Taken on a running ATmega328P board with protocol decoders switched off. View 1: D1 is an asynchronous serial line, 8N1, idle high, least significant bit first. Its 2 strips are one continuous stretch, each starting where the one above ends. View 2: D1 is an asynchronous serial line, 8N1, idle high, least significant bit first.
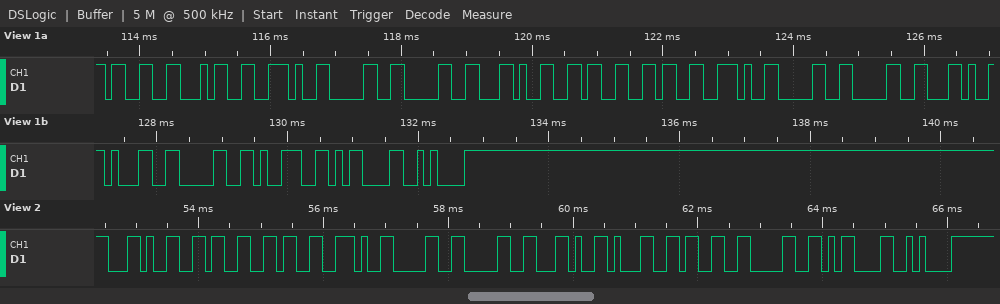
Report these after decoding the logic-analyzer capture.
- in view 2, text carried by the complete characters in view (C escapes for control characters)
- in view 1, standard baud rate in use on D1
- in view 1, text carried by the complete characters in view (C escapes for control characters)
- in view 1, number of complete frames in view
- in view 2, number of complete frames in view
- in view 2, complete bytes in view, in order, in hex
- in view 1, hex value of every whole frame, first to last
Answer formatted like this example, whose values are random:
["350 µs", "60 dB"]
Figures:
["\",66.00,130\\r\\n\"", "9600 baud", "\"34.00,66.00,109\\r\\n\"", "17", "12", "2C 36 36 2E 30 30 2C 31 33 30 0D 0A", "33 34 2E 30 30 2C 36 36 2E 30 30 2C 31 30 39 0D 0A"]
